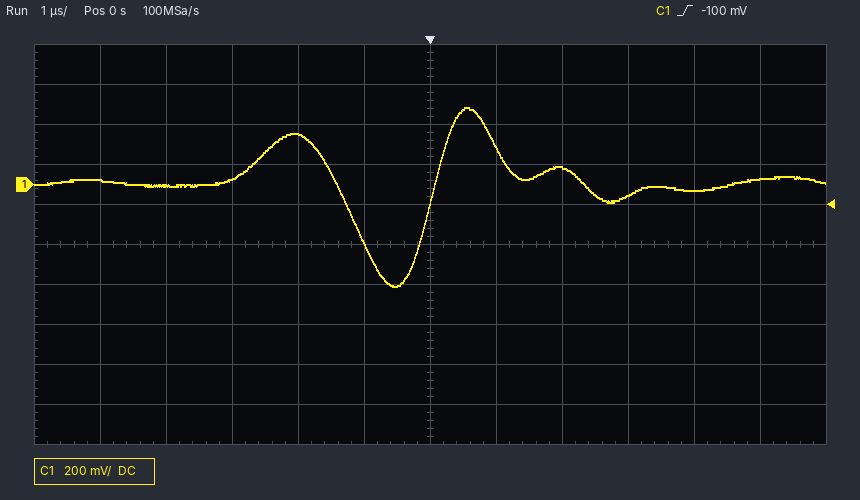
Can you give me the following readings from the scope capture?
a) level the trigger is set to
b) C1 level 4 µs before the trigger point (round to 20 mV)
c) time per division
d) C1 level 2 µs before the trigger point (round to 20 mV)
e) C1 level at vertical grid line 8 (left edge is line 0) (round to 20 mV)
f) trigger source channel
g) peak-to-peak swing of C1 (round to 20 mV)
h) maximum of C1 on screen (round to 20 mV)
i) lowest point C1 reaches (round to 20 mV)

-100 mV
0 mV
1 µs
260 mV
80 mV
C1
900 mV
380 mV
-520 mV
